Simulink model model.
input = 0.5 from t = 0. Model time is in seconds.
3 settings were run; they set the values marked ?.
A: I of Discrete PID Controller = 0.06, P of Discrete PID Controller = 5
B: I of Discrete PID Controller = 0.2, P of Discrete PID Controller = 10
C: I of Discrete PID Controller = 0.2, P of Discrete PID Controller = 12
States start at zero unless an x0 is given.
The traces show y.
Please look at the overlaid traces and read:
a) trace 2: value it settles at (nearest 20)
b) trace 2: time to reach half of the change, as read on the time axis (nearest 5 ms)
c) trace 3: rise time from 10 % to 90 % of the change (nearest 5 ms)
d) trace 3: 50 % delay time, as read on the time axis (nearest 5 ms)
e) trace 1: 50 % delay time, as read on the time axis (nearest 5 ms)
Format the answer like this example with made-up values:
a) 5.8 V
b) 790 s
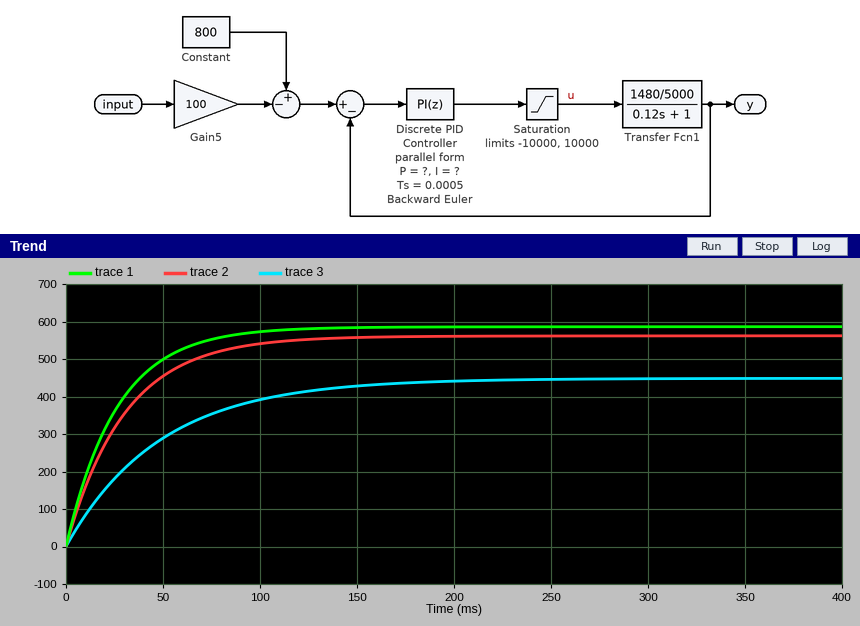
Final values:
a) 560
b) 20 ms
c) 110 ms
d) 35 ms
e) 20 ms
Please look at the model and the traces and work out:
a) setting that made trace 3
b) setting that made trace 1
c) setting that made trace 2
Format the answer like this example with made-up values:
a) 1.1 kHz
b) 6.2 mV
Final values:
a) A
b) C
c) B
